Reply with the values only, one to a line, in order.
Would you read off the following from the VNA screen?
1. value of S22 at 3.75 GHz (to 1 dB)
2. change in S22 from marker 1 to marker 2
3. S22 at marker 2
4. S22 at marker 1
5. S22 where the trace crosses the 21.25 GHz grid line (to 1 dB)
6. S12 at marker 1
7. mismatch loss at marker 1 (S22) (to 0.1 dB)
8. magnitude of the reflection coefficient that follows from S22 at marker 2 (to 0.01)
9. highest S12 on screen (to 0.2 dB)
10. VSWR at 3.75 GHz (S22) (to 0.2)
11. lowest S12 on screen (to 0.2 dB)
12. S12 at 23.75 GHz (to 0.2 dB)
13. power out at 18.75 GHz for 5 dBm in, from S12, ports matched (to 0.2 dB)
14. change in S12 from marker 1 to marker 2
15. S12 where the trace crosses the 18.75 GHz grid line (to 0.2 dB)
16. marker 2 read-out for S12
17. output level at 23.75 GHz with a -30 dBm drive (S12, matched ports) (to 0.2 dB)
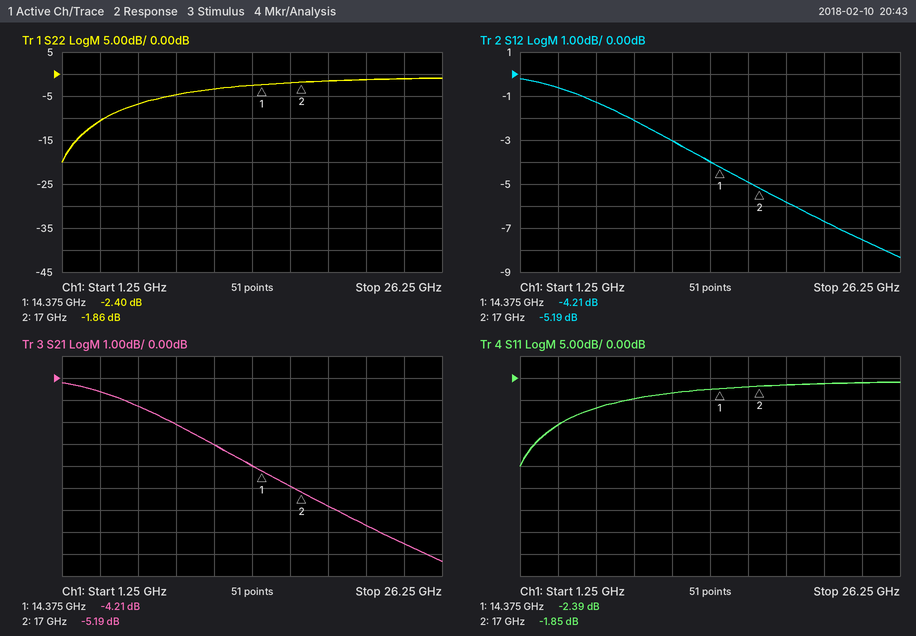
-11 dB
0.54 dB
-1.86 dB
-2.40 dB
-1 dB
-4.21 dB
3.7 dB
0.81
-0.2 dB
1.8
-8.4 dB
-7.6 dB
-0.8 dBm
-0.98 dB
-5.8 dB
-5.19 dB
-37.6 dBm
